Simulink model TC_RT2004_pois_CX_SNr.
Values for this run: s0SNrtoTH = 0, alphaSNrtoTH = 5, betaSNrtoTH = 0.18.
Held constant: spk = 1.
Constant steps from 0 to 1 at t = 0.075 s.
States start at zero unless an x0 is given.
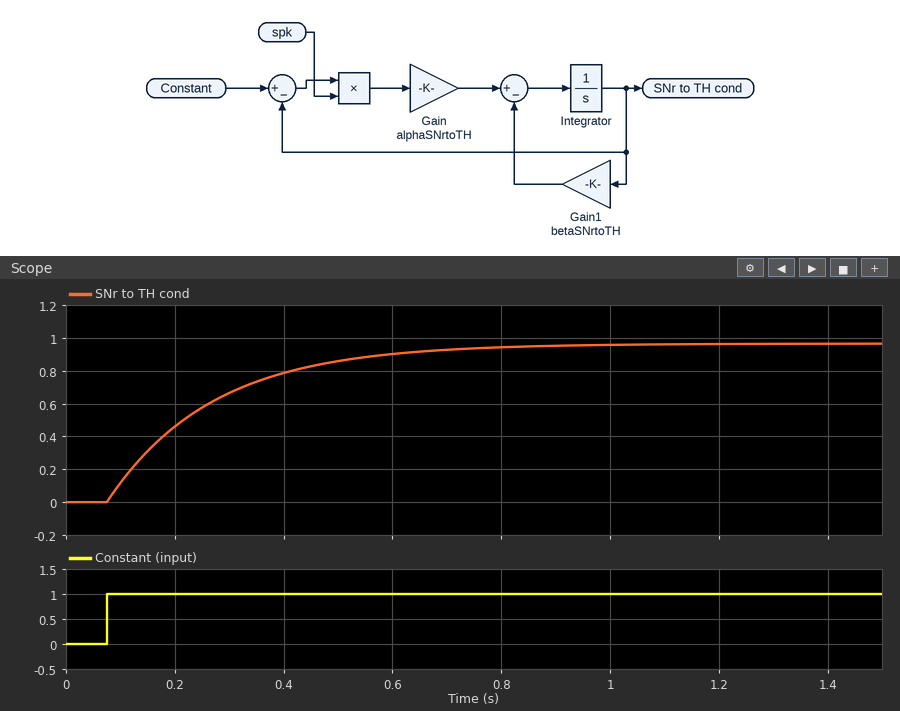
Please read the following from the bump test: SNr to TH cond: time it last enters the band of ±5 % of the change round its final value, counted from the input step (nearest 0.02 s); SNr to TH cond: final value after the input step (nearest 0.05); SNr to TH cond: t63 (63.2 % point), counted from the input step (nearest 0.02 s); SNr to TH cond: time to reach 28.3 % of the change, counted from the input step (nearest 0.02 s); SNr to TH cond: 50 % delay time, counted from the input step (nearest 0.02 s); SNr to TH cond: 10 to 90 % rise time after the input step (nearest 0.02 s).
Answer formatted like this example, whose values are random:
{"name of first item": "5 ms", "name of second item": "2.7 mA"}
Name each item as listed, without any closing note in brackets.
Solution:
{"SNr to TH cond: time it last enters the band of ±5 % of the change round its final value, counted from the input step": "0.58 s", "SNr to TH cond: final value after the input step": "0.95", "SNr to TH cond: t63 (63.2 % point), counted from the input step": "0.20 s", "SNr to TH cond: time to reach 28.3 % of the change, counted from the input step": "0.06 s", "SNr to TH cond: 50 % delay time, counted from the input step": "0.14 s", "SNr to TH cond: 10 to 90 % rise time after the input step": "0.42 s"}
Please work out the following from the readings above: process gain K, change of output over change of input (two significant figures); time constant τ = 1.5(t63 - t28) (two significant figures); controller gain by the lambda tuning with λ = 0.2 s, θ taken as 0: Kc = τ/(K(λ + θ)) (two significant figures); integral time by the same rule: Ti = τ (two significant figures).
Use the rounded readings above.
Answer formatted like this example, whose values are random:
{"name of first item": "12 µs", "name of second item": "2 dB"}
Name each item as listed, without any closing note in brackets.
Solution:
{"process gain K, change of output over change of input": "0.95", "time constant τ = 1.5(t63 - t28)": "0.21 s", "controller gain by the lambda tuning with λ = 0.2 s, θ taken as 0: Kc = τ/(K(λ + θ))": "1.1", "integral time by the same rule: Ti = τ": "0.21 s"}
